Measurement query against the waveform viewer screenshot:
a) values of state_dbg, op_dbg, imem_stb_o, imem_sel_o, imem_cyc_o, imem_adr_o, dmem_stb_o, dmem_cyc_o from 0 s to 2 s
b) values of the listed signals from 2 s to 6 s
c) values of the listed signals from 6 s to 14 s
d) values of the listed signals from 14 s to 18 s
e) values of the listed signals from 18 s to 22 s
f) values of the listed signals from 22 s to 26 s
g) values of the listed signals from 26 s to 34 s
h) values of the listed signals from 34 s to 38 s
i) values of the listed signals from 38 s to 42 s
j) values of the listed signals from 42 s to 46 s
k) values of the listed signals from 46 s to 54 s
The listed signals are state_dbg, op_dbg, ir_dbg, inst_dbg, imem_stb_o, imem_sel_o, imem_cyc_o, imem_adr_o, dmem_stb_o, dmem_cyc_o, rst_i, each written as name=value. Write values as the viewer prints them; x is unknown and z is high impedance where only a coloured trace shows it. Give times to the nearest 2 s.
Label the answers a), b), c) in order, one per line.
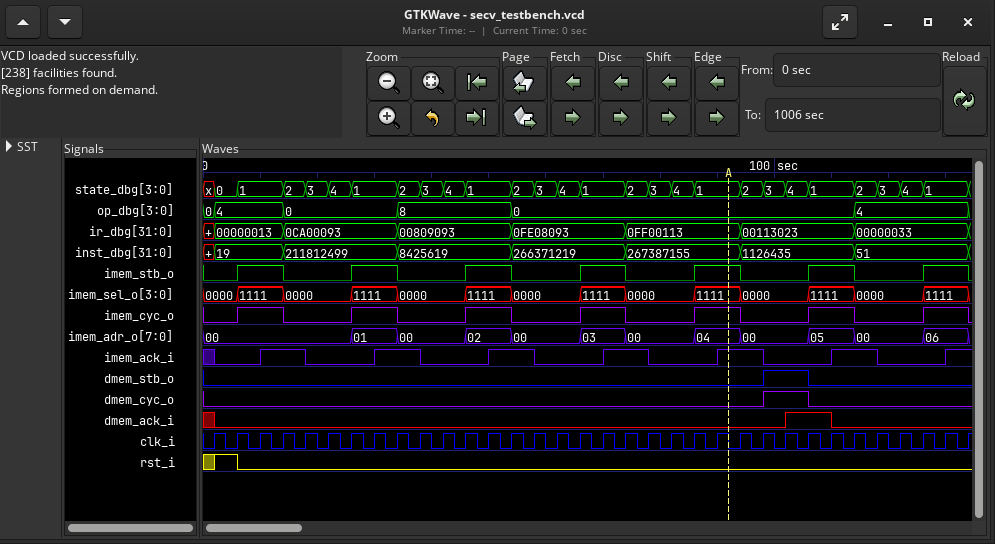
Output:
a) state_dbg=x, op_dbg=0, imem_stb_o=0, imem_sel_o=0000, imem_cyc_o=0, imem_adr_o=00, dmem_stb_o=0, dmem_cyc_o=0
b) state_dbg=0, op_dbg=4, ir_dbg=00000013, inst_dbg=19, imem_stb_o=0, imem_sel_o=0000, imem_cyc_o=0, imem_adr_o=00, dmem_stb_o=0, dmem_cyc_o=0, rst_i=1
c) state_dbg=1, op_dbg=4, ir_dbg=00000013, inst_dbg=19, imem_stb_o=1, imem_sel_o=1111, imem_cyc_o=1, imem_adr_o=00, dmem_stb_o=0, dmem_cyc_o=0, rst_i=0
d) state_dbg=2, op_dbg=0, ir_dbg=0CA00093, inst_dbg=211812499, imem_stb_o=0, imem_sel_o=0000, imem_cyc_o=0, imem_adr_o=00, dmem_stb_o=0, dmem_cyc_o=0, rst_i=0
e) state_dbg=3, op_dbg=0, ir_dbg=0CA00093, inst_dbg=211812499, imem_stb_o=0, imem_sel_o=0000, imem_cyc_o=0, imem_adr_o=00, dmem_stb_o=0, dmem_cyc_o=0, rst_i=0
f) state_dbg=4, op_dbg=0, ir_dbg=0CA00093, inst_dbg=211812499, imem_stb_o=0, imem_sel_o=0000, imem_cyc_o=0, imem_adr_o=00, dmem_stb_o=0, dmem_cyc_o=0, rst_i=0
g) state_dbg=1, op_dbg=0, ir_dbg=0CA00093, inst_dbg=211812499, imem_stb_o=1, imem_sel_o=1111, imem_cyc_o=1, imem_adr_o=01, dmem_stb_o=0, dmem_cyc_o=0, rst_i=0
h) state_dbg=2, op_dbg=8, ir_dbg=00809093, inst_dbg=8425619, imem_stb_o=0, imem_sel_o=0000, imem_cyc_o=0, imem_adr_o=00, dmem_stb_o=0, dmem_cyc_o=0, rst_i=0
i) state_dbg=3, op_dbg=8, ir_dbg=00809093, inst_dbg=8425619, imem_stb_o=0, imem_sel_o=0000, imem_cyc_o=0, imem_adr_o=00, dmem_stb_o=0, dmem_cyc_o=0, rst_i=0
j) state_dbg=4, op_dbg=8, ir_dbg=00809093, inst_dbg=8425619, imem_stb_o=0, imem_sel_o=0000, imem_cyc_o=0, imem_adr_o=00, dmem_stb_o=0, dmem_cyc_o=0, rst_i=0
k) state_dbg=1, op_dbg=8, ir_dbg=00809093, inst_dbg=8425619, imem_stb_o=1, imem_sel_o=1111, imem_cyc_o=1, imem_adr_o=02, dmem_stb_o=0, dmem_cyc_o=0, rst_i=0
